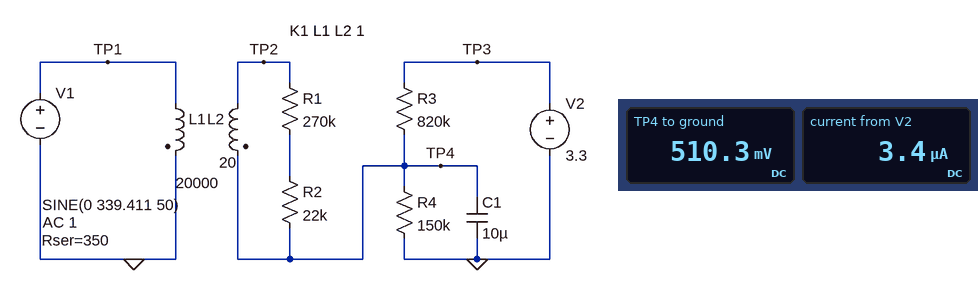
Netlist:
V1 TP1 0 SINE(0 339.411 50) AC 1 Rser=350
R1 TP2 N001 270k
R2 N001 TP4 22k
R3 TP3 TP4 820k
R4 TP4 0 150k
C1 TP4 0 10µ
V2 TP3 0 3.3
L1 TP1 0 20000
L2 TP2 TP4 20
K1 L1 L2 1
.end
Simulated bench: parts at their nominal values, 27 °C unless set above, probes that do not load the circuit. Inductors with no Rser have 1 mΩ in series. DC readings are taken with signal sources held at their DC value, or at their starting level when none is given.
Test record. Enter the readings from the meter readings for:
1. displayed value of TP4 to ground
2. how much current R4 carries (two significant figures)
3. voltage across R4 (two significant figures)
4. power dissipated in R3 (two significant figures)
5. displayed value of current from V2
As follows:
510.3 mV
3.4 µA
510 mV
9.5 µW
3.4 µA
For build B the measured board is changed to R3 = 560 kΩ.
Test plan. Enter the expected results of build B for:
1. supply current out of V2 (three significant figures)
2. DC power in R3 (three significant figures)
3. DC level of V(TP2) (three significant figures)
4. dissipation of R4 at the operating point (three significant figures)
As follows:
4.65 µA
12.1 µW
697 mV
3.24 µW
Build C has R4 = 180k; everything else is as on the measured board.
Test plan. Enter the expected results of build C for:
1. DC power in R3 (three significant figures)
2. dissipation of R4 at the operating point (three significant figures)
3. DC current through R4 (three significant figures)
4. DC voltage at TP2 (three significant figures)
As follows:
8.93 µW
1.96 µW
3.30 µA
594 mV
